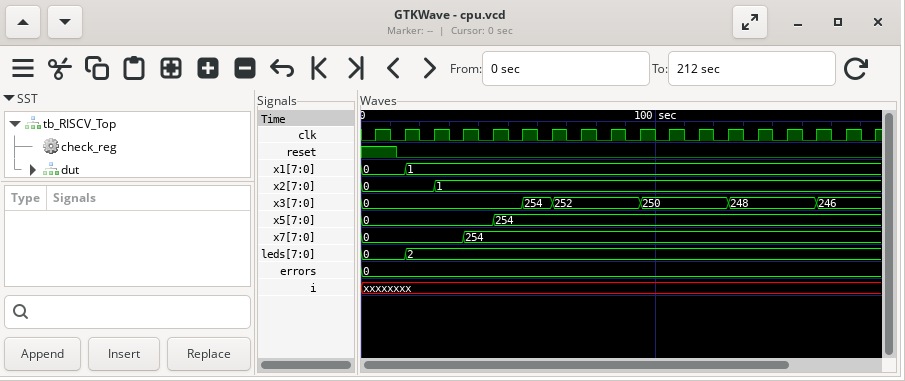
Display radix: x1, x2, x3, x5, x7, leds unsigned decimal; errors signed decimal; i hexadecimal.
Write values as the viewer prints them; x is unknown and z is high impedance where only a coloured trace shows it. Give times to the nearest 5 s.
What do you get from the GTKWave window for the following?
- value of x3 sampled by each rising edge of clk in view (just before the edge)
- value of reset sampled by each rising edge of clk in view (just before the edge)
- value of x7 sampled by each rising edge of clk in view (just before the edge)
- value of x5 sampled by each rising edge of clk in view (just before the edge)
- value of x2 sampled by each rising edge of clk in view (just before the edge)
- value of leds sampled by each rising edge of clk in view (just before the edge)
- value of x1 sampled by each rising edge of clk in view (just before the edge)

0, 0, 0, 0, 0, 0, 254, 252, 252, 252, 250, 250, 250, 248, 248, 248, 246, 246
1 0 0 0 0 0 0 0 0 0 0 0 0 0 0 0 0 0
0, 0, 0, 0, 254, 254, 254, 254, 254, 254, 254, 254, 254, 254, 254, 254, 254, 254
0, 0, 0, 0, 0, 254, 254, 254, 254, 254, 254, 254, 254, 254, 254, 254, 254, 254
0, 0, 0, 1, 1, 1, 1, 1, 1, 1, 1, 1, 1, 1, 1, 1, 1, 1
0, 0, 2, 2, 2, 2, 2, 2, 2, 2, 2, 2, 2, 2, 2, 2, 2, 2
0, 0, 1, 1, 1, 1, 1, 1, 1, 1, 1, 1, 1, 1, 1, 1, 1, 1
